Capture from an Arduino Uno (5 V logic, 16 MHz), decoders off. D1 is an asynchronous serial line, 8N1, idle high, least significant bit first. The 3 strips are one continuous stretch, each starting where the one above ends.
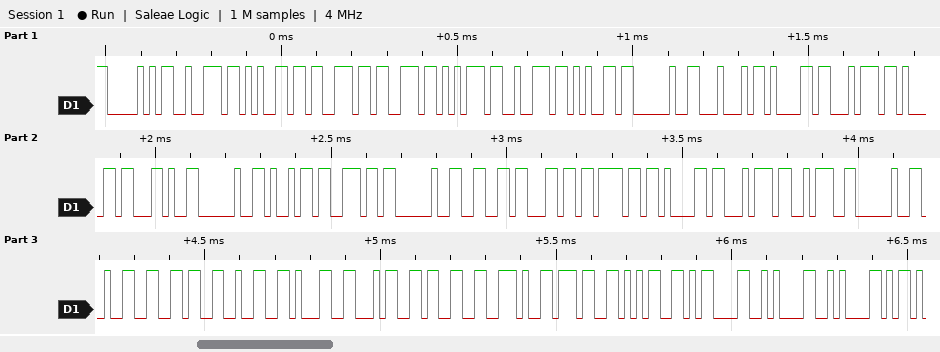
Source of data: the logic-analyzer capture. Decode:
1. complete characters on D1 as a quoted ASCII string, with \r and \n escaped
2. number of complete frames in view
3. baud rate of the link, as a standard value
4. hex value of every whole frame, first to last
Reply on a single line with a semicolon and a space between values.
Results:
"Pressure Data, in float: 262143.75\r\n\n"; 37; 57600 baud; 50 72 65 73 73 75 72 65 20 44 61 74 61 2C 20 69 6E 20 66 6C 6F 61 74 3A 20 32 36 32 31 34 33 2E 37 35 0D 0A 0A
